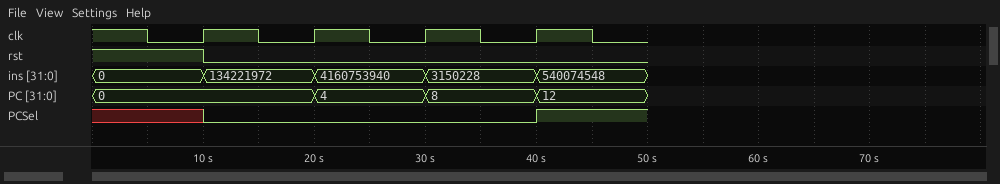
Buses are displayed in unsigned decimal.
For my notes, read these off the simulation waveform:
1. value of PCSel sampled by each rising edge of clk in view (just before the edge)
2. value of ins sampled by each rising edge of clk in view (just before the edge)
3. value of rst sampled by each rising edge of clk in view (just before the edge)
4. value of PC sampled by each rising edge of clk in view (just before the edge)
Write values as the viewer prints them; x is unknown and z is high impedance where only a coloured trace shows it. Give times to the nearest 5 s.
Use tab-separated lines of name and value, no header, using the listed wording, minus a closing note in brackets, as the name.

value of PCSel sampled by each rising edge of clk in view	x 0 0 0
value of ins sampled by each rising edge of clk in view	0, 134221972, 4160753940, 3150228
value of rst sampled by each rising edge of clk in view	1 0 0 0
value of PC sampled by each rising edge of clk in view	0, 0, 4, 8
